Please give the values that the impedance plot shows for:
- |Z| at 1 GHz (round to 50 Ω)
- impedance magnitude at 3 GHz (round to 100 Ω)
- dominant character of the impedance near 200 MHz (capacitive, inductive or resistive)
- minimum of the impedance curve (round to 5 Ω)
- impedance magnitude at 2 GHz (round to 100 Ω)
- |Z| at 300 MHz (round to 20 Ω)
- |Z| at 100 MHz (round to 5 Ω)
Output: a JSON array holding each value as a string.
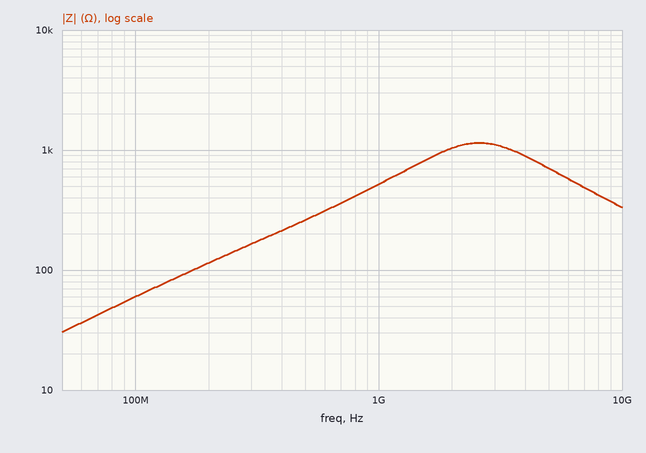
["500 Ω", "1.1 kΩ", "inductive", "30 Ω", "1.0 kΩ", "160 Ω", "60 Ω"]
